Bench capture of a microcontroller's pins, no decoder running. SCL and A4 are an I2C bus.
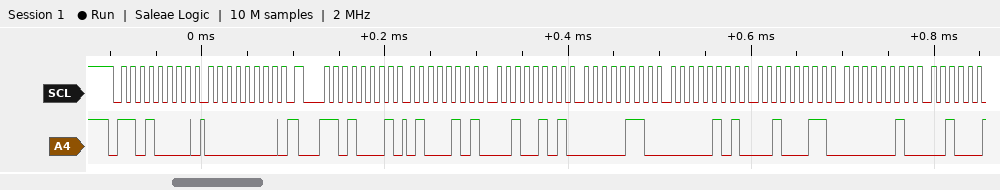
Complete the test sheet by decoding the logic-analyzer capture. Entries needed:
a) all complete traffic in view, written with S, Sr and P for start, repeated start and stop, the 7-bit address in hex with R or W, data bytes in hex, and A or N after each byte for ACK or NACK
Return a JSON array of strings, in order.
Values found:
["S 68W A 00 A Sr 68R A 45 A 25 A 06 A 05 A 23 A 02 A"]
